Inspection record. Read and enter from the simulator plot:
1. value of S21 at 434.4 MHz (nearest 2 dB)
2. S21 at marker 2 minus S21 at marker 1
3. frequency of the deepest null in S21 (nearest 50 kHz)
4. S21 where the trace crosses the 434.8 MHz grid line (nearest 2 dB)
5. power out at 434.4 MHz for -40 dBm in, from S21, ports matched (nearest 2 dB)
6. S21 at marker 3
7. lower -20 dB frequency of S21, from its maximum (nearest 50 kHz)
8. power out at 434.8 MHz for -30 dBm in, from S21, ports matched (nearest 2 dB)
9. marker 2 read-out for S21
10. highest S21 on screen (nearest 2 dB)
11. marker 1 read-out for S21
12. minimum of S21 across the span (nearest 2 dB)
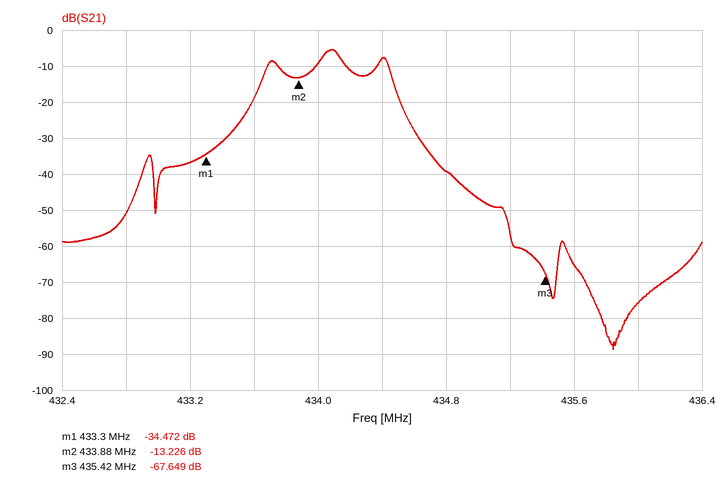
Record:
-8 dB
21.246 dB
435.85 MHz
-40 dB
-48 dBm
-67.649 dB
433.50 MHz
-70 dBm
-13.226 dB
-6 dB
-34.472 dB
-88 dB
